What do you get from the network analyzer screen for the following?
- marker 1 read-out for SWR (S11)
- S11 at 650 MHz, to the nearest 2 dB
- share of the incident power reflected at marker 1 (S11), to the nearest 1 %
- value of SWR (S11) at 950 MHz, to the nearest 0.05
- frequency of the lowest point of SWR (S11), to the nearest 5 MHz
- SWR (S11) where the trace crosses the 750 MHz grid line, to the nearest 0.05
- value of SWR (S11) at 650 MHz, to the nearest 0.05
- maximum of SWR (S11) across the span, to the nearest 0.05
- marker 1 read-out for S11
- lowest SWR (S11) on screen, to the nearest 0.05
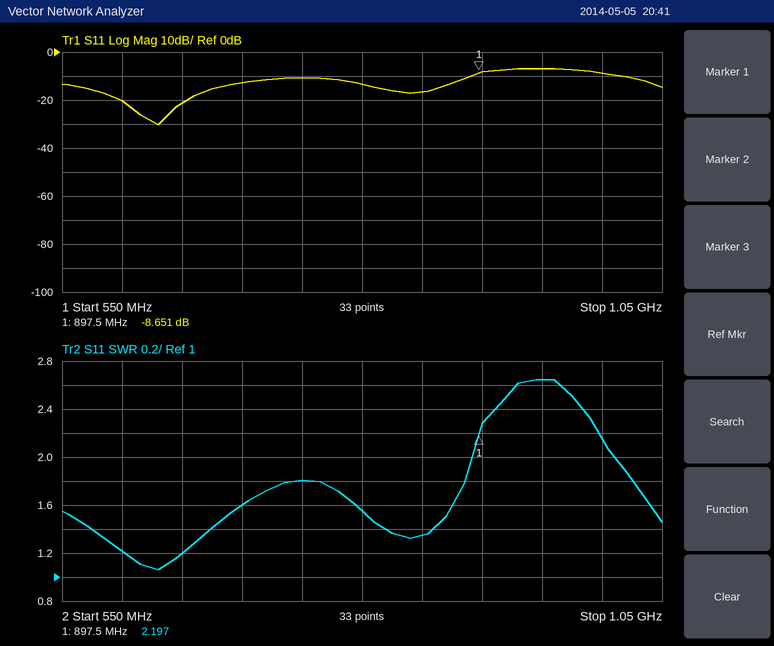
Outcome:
2.197
-22 dB
14 %
2.65
630 MHz
1.80
1.20
2.65
-8.651 dB
1.05
